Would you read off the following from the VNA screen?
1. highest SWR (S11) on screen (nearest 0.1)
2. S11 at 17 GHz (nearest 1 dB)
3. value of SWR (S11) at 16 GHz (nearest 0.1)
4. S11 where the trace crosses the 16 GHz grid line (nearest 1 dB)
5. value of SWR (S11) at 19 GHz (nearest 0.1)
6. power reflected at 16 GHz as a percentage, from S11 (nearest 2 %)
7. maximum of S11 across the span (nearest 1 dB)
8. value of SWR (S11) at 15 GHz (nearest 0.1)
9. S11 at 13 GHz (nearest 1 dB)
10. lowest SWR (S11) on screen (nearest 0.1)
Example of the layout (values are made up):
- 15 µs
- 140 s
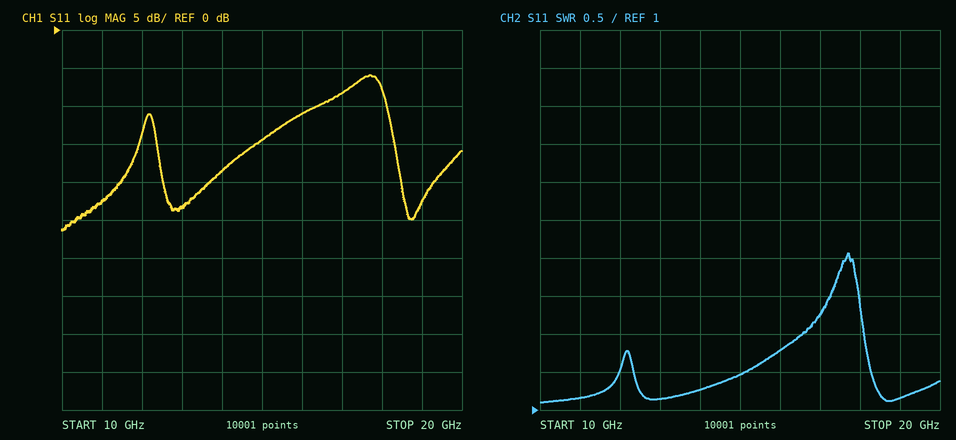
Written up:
- 3.1
- -8 dB
- 1.8
- -11 dB
- 1.2
- 8 %
- -6 dB
- 1.5
- -23 dB
- 1.1
